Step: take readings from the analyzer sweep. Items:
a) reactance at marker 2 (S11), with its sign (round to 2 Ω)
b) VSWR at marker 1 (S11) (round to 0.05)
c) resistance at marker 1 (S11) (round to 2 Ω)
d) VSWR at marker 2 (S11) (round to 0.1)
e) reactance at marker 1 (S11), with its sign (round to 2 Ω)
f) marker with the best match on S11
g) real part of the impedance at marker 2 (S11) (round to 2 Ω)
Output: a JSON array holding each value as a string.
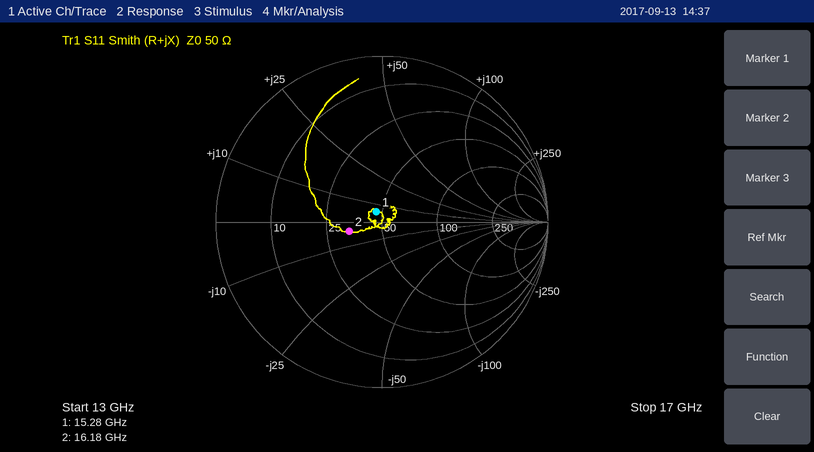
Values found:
["-4 Ω", "1.15", "46 Ω", "1.5", "+6 Ω", "marker 1", "34 Ω"]
